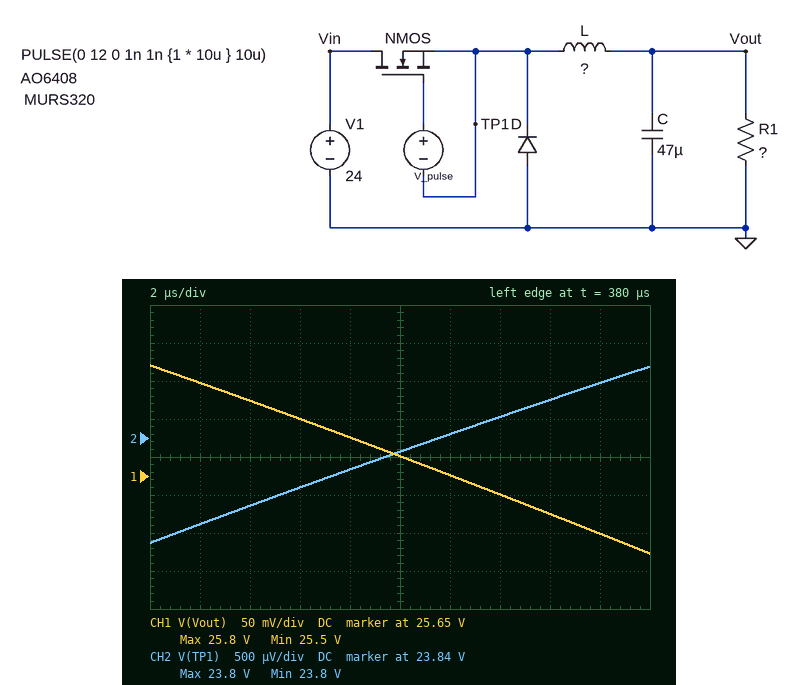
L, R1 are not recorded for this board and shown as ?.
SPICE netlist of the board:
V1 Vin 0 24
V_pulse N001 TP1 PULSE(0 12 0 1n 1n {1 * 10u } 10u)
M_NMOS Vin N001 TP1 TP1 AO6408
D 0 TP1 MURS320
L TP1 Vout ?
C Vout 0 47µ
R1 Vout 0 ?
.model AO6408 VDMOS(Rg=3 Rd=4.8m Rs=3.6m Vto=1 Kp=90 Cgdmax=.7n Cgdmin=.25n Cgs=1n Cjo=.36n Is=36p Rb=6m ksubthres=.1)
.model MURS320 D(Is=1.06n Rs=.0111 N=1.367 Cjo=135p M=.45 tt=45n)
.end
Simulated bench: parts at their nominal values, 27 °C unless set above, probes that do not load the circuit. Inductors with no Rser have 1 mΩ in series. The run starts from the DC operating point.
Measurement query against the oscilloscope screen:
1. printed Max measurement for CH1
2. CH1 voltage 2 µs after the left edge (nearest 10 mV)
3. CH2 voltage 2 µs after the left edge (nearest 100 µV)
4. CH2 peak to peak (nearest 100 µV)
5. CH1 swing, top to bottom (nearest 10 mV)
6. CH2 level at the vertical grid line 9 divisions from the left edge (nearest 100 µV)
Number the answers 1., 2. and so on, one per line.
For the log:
1. 25.8 V
2. 25.77 V
3. 23.8434 V
4. 2.3 mV
5. 250 mV
6. 23.8452 V
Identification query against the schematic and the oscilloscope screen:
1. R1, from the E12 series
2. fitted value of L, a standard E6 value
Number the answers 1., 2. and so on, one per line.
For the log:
1. 1.5 Ω
2. 150 µH
